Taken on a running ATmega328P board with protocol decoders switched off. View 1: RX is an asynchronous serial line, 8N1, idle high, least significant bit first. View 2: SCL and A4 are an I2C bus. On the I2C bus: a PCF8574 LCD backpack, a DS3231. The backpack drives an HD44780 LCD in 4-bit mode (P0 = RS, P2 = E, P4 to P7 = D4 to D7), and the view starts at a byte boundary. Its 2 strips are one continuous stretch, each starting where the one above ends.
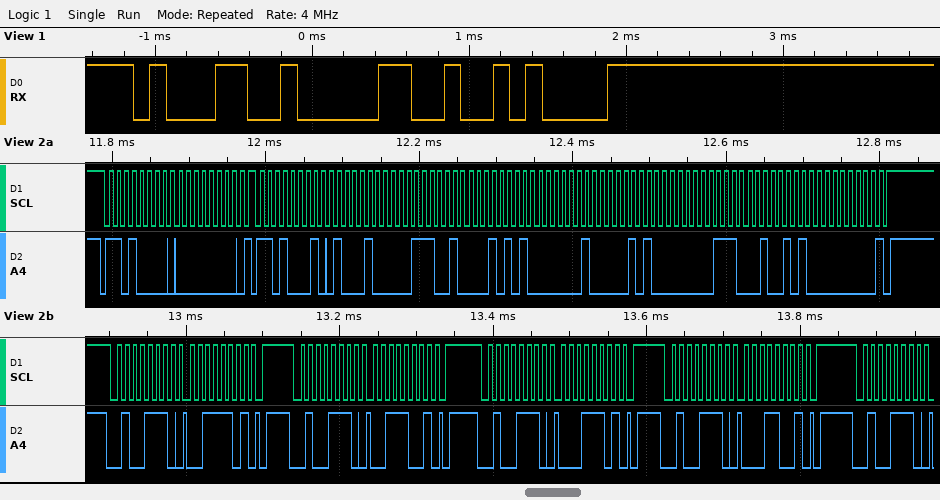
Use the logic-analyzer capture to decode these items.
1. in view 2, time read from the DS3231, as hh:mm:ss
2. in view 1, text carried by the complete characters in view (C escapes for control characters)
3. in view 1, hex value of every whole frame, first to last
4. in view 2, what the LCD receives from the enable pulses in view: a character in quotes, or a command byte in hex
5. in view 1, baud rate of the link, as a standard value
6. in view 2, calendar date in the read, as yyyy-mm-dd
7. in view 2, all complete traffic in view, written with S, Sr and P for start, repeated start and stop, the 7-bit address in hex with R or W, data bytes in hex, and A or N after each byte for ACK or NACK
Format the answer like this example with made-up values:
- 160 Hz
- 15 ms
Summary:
- 15:39:44
- "10\n"
- 0x31 0x30 0x0A
- '1'
- 9600 baud
- 2025-07-14
- S 68W A 00 A Sr 68R A 44 A 39 A 15 A 02 A 14 A 07 A 25 A 00 N P S 27W A 3D A P S 27W A 39 A P S 27W A 1D A P S 27W A 19 A P S 27W A
